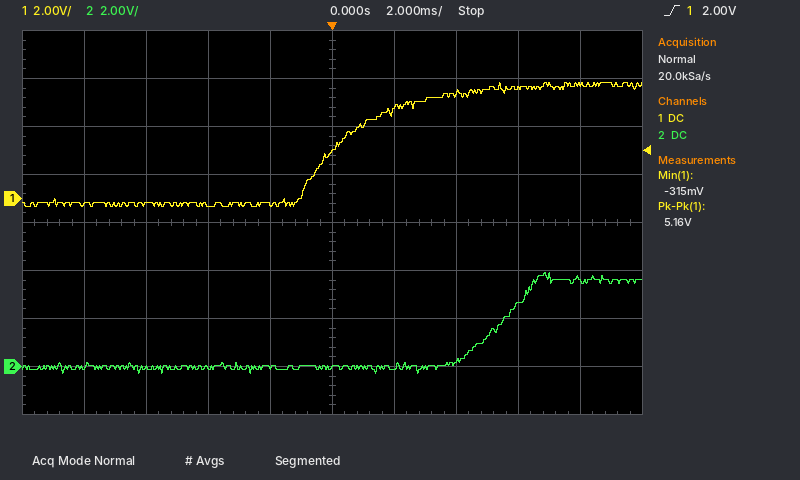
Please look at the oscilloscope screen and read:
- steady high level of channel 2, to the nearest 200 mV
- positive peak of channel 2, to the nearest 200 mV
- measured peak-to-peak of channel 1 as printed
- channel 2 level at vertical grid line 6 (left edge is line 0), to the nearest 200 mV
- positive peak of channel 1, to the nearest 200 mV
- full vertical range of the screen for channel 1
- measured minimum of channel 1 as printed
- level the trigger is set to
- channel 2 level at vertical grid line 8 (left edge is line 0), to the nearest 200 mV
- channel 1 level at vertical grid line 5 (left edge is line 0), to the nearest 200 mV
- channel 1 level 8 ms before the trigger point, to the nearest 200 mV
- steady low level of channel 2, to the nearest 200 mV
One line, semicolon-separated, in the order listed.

3.6 V; 4.0 V; 5.16 V; 0.0 V; 4.8 V; 16 V; -315 mV; 2.00 V; 2.6 V; 2.0 V; -200 mV; 0.0 V
